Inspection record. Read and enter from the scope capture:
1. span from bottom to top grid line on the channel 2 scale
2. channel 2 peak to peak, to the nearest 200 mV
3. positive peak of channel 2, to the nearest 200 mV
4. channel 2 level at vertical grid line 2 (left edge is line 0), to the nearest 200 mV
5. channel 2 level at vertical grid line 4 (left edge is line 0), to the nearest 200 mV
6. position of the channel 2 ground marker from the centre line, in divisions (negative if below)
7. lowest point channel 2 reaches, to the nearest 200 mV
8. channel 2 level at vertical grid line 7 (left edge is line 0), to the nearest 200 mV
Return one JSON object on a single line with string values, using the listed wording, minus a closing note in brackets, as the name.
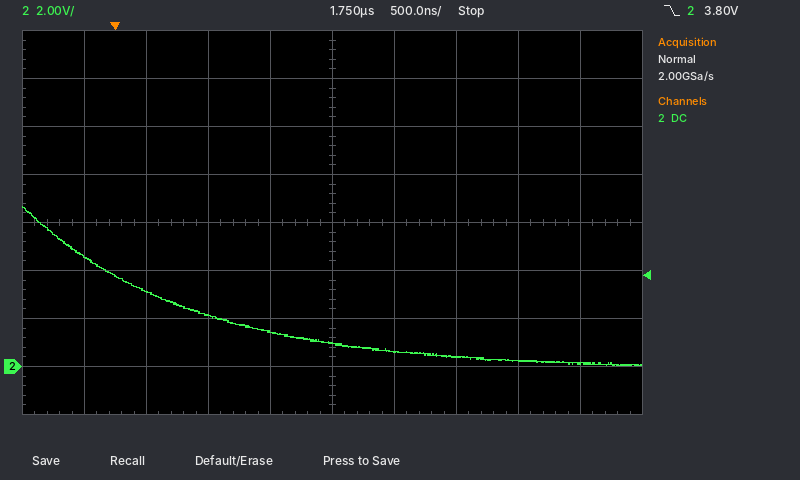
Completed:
{"span from bottom to top grid line on the channel 2 scale": "16 V", "channel 2 peak to peak, to the nearest 200 mV": "6.6 V", "positive peak of channel 2, to the nearest 200 mV": "6.6 V", "channel 2 level at vertical grid line 2 (left edge is line 0), to the nearest 200 mV": "3.2 V", "channel 2 level at vertical grid line 4 (left edge is line 0), to the nearest 200 mV": "1.4 V", "position of the channel 2 ground marker from the centre line, in divisions": "-3.0 div", "lowest point channel 2 reaches, to the nearest 200 mV": "0.0 V", "channel 2 level at vertical grid line 7 (left edge is line 0), to the nearest 200 mV": "400 mV"}
